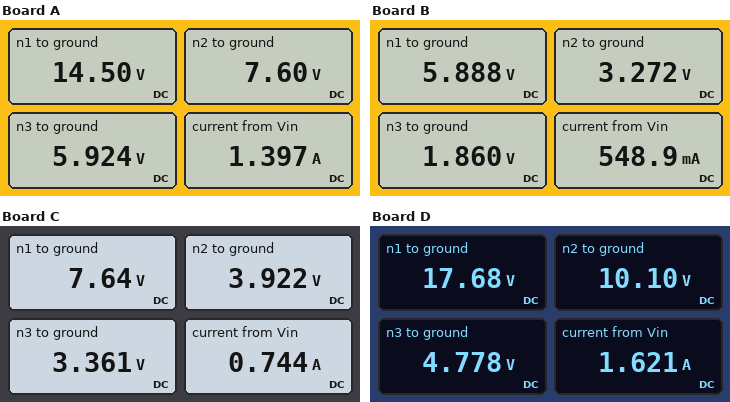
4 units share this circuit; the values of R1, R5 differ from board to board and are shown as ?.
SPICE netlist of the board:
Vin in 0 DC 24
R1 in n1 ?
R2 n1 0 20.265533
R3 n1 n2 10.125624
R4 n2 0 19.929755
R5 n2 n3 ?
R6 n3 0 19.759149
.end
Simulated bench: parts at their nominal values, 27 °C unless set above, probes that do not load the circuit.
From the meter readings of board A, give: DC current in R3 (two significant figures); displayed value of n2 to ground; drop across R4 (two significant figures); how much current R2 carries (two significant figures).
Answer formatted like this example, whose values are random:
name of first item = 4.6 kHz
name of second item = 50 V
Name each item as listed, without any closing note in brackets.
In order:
DC current in R3 = 680 mA
displayed value of n2 to ground = 7.60 V
drop across R4 = 7.6 V
how much current R2 carries = 720 mA
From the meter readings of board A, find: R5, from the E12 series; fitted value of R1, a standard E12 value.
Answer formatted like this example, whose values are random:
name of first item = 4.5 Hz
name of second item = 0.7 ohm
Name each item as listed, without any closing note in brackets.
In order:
R5, from the E12 series = 5.6 Ω
fitted value of R1, a standard E12 value = 6.8 Ω
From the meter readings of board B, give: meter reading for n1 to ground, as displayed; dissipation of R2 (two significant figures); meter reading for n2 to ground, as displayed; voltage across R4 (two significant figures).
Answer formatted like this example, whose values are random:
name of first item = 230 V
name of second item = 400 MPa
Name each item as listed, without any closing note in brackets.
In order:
meter reading for n1 to ground, as displayed = 5.888 V
dissipation of R2 = 1.7 W
meter reading for n2 to ground, as displayed = 3.272 V
voltage across R4 = 3.3 V
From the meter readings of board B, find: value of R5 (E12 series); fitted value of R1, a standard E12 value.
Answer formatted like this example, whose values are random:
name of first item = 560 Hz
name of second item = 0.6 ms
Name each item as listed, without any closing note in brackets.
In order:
value of R5 = 15 Ω
fitted value of R1, a standard E12 value = 33 Ω
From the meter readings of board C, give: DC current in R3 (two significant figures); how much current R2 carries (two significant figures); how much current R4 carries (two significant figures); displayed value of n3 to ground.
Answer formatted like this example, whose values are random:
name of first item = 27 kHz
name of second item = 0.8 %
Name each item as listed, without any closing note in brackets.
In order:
DC current in R3 = 370 mA
how much current R2 carries = 380 mA
how much current R4 carries = 200 mA
displayed value of n3 to ground = 3.361 V
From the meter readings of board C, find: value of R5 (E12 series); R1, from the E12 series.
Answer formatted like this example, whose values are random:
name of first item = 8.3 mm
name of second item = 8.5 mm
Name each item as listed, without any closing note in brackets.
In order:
value of R5 = 3.3 Ω
R1, from the E12 series = 22 Ω
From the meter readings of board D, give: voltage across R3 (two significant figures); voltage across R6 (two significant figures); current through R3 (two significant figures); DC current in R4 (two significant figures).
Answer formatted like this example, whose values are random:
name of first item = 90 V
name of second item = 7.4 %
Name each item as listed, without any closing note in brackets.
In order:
voltage across R3 = 7.6 V
voltage across R6 = 4.8 V
current through R3 = 750 mA
DC current in R4 = 510 mA
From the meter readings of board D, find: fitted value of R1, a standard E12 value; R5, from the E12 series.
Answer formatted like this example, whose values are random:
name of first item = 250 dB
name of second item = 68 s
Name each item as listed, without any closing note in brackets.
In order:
fitted value of R1, a standard E12 value = 3.9 Ω
R5, from the E12 series = 22 Ω
